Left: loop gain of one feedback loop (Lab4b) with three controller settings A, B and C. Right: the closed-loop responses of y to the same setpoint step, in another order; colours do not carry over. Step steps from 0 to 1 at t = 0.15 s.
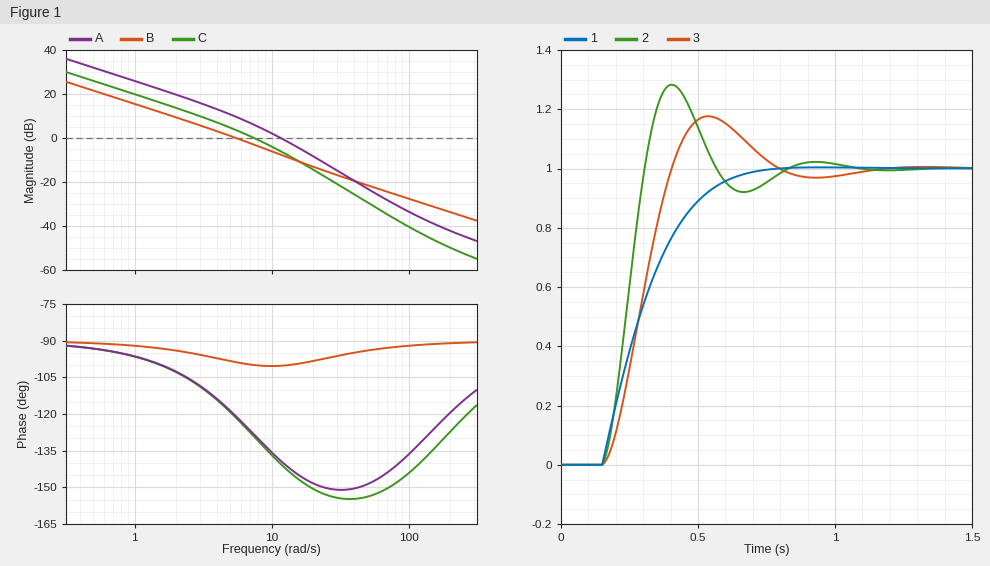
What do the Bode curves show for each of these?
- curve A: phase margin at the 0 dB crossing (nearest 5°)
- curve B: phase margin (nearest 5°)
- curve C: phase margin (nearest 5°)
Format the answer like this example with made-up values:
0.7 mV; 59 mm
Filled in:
40°; 80°; 50°
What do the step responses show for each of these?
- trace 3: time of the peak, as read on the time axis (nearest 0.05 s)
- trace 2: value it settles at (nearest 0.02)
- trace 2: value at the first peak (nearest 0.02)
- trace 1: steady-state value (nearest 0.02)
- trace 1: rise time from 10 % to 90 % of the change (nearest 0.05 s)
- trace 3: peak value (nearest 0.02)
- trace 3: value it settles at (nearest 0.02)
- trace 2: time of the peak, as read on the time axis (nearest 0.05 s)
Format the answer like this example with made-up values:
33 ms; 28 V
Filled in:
0.55 s; 1.00; 1.28; 1.00; 0.35 s; 1.18; 1.00; 0.40 s
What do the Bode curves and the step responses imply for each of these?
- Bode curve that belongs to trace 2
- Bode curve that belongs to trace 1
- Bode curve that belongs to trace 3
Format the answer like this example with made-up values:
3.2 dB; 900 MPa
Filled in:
A; B; C
